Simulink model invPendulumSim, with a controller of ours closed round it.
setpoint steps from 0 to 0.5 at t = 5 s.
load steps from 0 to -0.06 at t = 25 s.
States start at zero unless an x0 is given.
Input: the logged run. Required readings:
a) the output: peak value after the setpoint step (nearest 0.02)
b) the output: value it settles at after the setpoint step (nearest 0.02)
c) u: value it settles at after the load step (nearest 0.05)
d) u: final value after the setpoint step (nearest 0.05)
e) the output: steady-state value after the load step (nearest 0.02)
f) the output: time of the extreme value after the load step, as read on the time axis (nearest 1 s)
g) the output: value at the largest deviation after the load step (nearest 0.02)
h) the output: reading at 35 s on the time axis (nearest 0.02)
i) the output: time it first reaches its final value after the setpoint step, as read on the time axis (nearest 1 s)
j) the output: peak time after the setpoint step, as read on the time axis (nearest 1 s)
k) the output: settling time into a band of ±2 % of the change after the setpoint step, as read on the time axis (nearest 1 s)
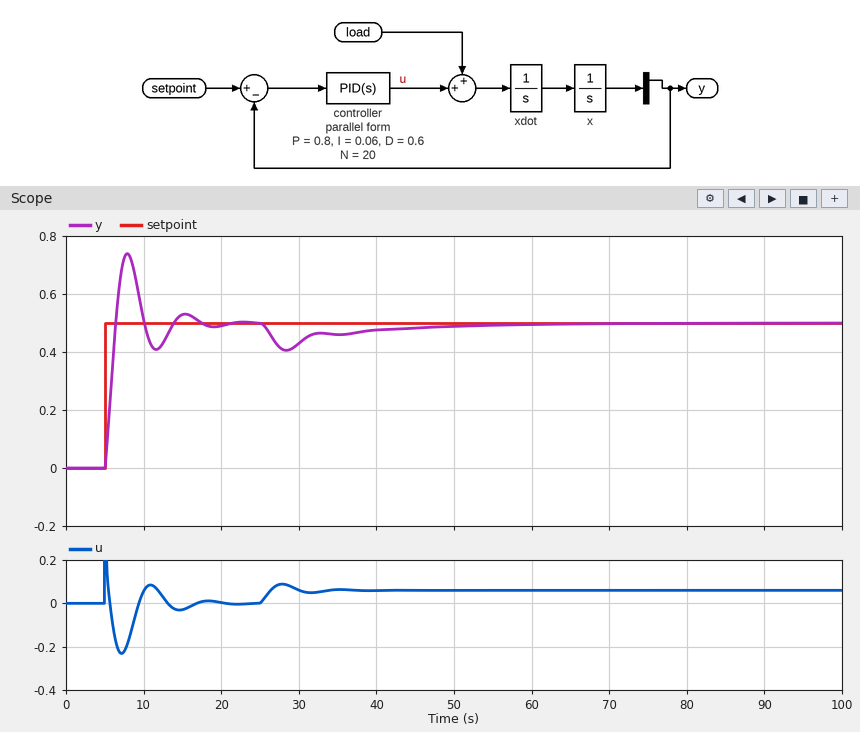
0.74
0.50
0.05
0.00
0.50
28 s
0.40
0.46
6 s
8 s
20 s
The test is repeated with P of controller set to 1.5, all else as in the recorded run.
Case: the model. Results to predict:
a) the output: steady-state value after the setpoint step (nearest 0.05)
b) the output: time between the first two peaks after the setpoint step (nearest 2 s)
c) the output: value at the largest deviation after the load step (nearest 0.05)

0.50
6 s
0.45
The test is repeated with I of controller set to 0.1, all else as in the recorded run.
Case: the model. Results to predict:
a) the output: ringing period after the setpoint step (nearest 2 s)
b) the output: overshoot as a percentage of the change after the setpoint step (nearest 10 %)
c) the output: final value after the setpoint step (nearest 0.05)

8 s
50 %
0.50
